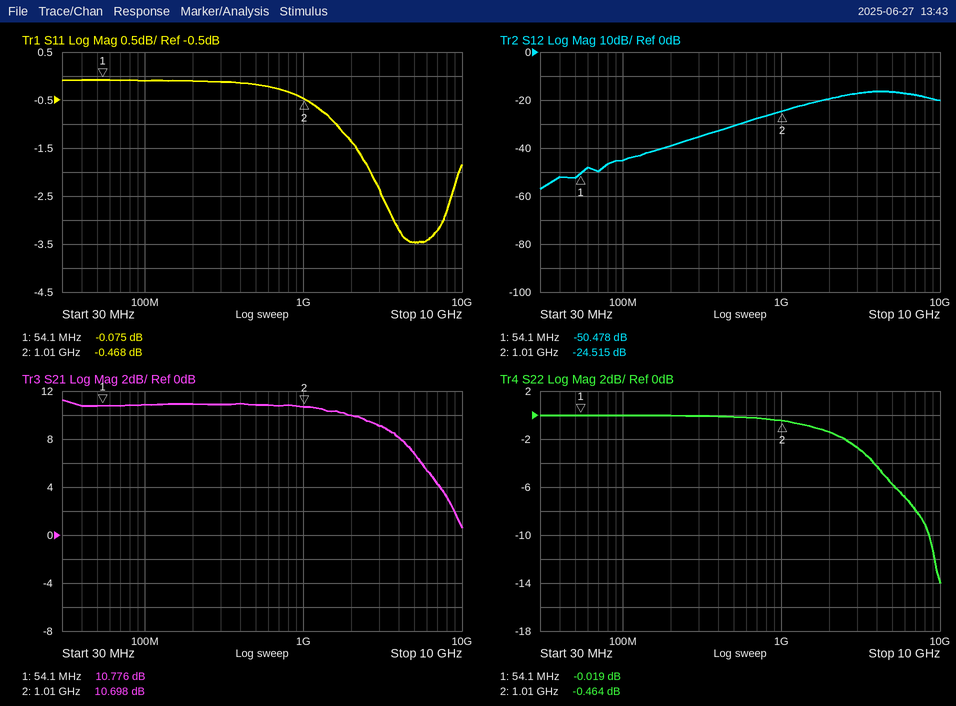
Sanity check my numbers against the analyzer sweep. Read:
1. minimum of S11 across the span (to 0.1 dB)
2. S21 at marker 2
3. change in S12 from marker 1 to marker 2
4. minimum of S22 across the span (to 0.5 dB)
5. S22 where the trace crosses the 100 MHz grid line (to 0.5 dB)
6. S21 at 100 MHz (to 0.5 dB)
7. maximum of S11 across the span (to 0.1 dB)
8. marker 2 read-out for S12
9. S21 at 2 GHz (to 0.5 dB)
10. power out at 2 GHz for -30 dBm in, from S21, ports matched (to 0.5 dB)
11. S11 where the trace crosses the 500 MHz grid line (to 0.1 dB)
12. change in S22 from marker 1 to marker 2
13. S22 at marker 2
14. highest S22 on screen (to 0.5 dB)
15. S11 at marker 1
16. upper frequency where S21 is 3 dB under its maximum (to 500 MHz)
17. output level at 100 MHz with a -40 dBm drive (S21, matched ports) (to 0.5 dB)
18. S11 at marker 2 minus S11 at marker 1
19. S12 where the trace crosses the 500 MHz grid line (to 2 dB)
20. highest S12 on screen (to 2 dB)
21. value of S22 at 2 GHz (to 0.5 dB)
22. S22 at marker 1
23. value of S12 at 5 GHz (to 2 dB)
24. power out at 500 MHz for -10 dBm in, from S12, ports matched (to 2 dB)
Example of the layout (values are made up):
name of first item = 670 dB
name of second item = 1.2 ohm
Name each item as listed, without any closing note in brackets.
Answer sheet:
minimum of S11 across the span = -3.5 dB
S21 at marker 2 = 10.698 dB
change in S12 from marker 1 to marker 2 = 25.963 dB
minimum of S22 across the span = -14.0 dB
S22 where the trace crosses the 100 MHz grid line = 0.0 dB
S21 at 100 MHz = 11.0 dB
maximum of S11 across the span = -0.1 dB
marker 2 read-out for S12 = -24.515 dB
S21 at 2 GHz = 10.0 dB
power out at 2 GHz for -30 dBm in, from S21, ports matched = -20.0 dBm
S11 where the trace crosses the 500 MHz grid line = -0.2 dB
change in S22 from marker 1 to marker 2 = -0.445 dB
S22 at marker 2 = -0.464 dB
highest S22 on screen = 0.0 dB
S11 at marker 1 = -0.075 dB
upper frequency where S21 is 3 dB under its maximum = 4.0 GHz
output level at 100 MHz with a -40 dBm drive (S21, matched ports) = -29.0 dBm
S11 at marker 2 minus S11 at marker 1 = -0.393 dB
S12 where the trace crosses the 500 MHz grid line = -30 dB
highest S12 on screen = -16 dB
value of S22 at 2 GHz = -1.5 dB
S22 at marker 1 = -0.019 dB
value of S12 at 5 GHz = -16 dB
power out at 500 MHz for -10 dBm in, from S12, ports matched = -40 dBm
